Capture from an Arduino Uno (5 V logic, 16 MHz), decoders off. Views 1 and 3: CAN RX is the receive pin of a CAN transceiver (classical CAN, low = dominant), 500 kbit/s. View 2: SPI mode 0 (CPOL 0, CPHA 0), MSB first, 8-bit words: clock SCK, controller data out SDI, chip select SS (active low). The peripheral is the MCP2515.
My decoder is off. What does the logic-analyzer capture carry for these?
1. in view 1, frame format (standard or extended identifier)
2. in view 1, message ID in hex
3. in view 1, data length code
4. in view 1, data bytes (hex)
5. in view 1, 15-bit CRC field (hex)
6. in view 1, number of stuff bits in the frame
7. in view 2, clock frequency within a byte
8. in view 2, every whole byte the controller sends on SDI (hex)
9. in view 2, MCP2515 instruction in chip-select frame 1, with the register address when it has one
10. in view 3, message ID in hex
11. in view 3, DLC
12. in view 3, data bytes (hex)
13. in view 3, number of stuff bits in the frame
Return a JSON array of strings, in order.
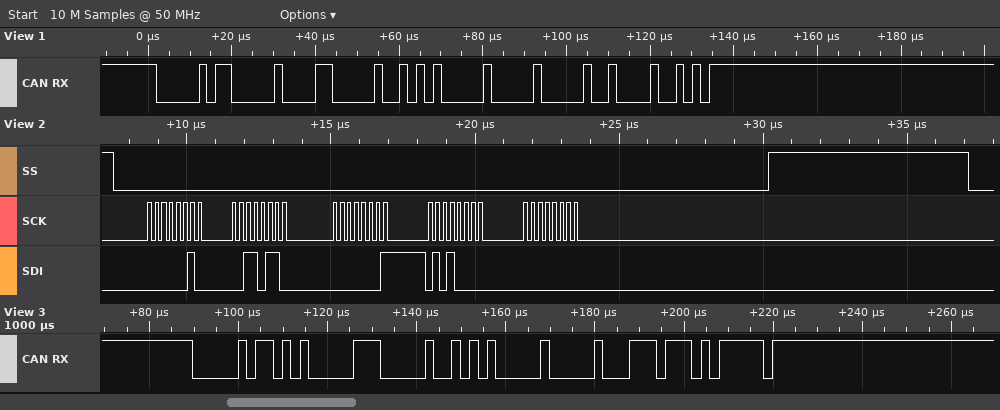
["standard", "0x030", "3", "01 50 00", "0x0212", "6", "4 MHz", "02 36 01 50 00", "WRITE 0x36", "0x035", "3", "01 50 00", "5"]
